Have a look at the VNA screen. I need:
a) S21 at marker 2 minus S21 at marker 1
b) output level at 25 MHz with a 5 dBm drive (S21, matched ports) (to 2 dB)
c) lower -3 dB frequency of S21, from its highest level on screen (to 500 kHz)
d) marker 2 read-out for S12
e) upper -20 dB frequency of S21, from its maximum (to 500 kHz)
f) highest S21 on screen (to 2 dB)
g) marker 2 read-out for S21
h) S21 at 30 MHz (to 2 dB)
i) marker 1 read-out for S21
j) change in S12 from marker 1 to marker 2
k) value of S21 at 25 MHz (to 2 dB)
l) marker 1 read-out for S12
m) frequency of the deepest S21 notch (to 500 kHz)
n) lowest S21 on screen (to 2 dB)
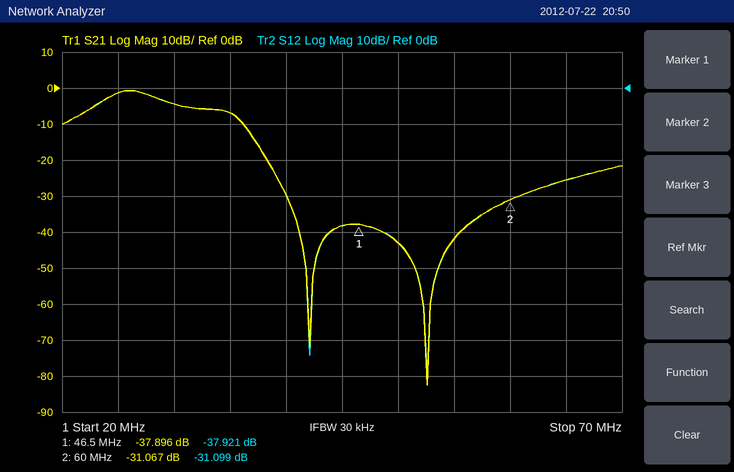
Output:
6.829 dB
4 dBm
23.5 MHz
-31.099 dB
38.5 MHz
0 dB
-31.067 dB
-4 dB
-37.896 dB
6.822 dB
-2 dB
-37.921 dB
52.5 MHz
-82 dB
